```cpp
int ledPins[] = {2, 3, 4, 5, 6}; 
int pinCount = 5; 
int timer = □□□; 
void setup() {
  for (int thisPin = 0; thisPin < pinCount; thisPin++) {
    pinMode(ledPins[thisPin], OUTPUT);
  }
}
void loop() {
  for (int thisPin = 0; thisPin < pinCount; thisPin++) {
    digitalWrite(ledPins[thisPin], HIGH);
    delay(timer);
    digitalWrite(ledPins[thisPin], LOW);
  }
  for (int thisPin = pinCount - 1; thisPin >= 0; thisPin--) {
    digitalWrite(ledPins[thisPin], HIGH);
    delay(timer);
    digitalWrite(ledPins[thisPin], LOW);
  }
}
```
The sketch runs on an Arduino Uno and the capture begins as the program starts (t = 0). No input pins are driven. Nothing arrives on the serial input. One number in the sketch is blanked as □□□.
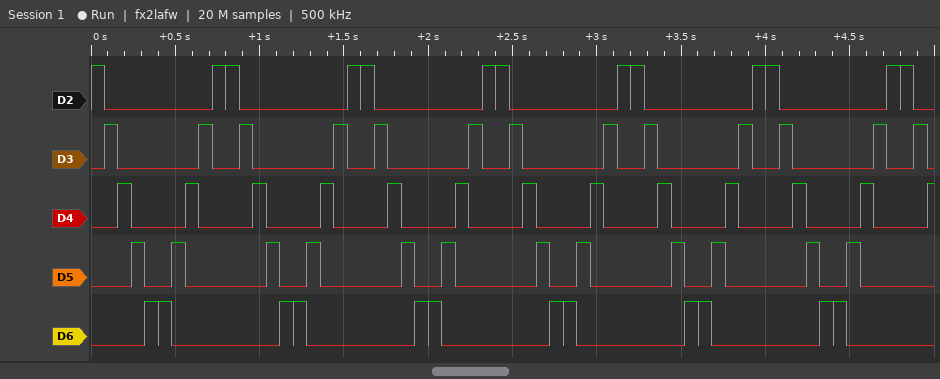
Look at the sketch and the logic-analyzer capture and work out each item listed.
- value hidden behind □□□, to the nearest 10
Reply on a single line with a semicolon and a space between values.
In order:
80
